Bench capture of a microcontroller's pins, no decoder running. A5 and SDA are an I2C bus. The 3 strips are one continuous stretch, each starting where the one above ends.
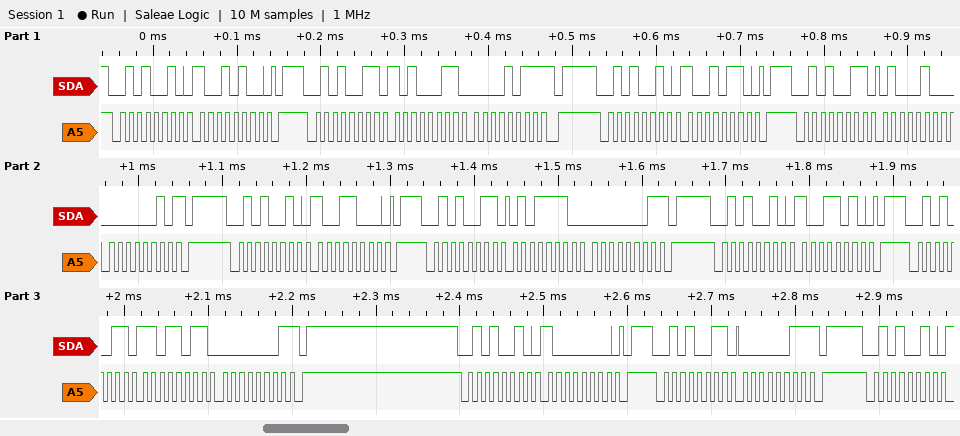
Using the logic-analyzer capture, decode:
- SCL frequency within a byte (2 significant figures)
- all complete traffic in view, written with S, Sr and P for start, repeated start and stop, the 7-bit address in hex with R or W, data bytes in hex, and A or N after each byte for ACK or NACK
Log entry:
100 kHz
S 29W A 94 A P S 29R A A3 A 0B N P S 29W A 96 A P S 29R A 44 A 02 N P S 29W A 98 A P S 29R A 5E A 01 N P S 29W A 9A A P S 29R A DB A 01 N P S 29W A 80 A P S 29R A 03 N P S 29W A
